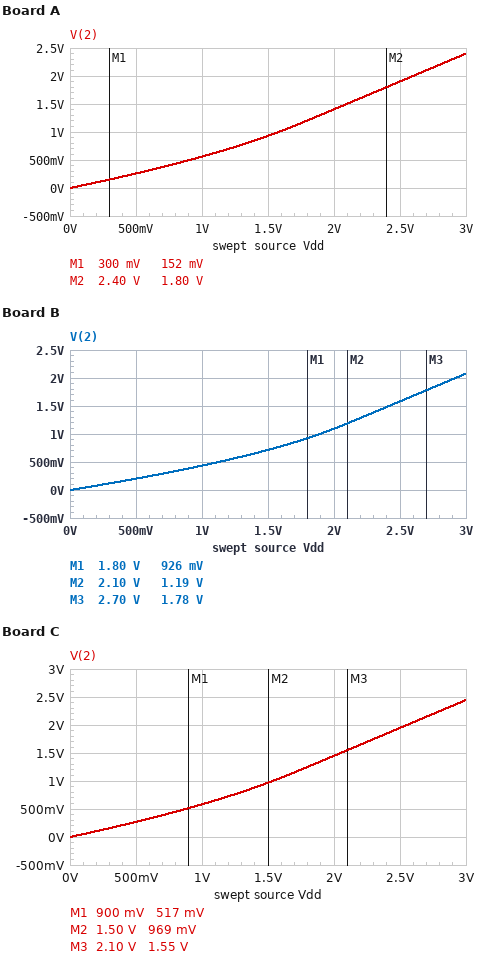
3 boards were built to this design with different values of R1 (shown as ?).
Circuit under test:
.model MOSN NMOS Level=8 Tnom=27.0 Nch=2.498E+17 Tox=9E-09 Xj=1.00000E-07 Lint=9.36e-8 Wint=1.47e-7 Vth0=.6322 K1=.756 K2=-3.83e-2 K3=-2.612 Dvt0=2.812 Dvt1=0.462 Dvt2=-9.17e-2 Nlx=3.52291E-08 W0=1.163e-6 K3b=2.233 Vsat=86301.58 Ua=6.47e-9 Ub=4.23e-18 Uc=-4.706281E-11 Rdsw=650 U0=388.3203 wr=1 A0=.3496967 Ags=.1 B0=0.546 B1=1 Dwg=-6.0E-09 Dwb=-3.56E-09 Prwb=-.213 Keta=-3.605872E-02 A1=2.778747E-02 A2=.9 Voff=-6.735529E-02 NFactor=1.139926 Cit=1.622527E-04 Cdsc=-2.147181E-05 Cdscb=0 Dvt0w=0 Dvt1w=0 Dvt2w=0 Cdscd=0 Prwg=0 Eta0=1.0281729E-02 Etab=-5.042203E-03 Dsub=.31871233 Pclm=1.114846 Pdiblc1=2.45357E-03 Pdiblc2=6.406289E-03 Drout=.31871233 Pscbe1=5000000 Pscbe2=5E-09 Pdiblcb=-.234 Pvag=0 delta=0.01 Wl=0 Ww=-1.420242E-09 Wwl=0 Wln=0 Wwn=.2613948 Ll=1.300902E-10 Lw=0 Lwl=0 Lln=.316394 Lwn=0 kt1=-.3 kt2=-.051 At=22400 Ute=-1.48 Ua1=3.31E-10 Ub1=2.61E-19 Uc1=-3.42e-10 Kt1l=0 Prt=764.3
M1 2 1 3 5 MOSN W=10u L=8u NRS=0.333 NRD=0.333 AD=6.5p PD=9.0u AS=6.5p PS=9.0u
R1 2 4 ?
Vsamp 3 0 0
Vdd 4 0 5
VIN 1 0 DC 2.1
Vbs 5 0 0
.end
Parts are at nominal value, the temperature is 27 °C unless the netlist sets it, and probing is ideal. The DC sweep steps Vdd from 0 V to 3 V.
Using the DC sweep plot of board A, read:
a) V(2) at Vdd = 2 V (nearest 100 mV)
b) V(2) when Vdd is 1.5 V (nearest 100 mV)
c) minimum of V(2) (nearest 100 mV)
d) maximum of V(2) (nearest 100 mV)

1.4 V
900 mV
0 V
2.4 V
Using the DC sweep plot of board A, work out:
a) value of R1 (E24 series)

13 kΩ
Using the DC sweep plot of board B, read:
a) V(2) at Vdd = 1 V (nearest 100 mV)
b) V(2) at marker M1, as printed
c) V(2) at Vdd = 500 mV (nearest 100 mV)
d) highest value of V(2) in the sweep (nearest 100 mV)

400 mV
926 mV
200 mV
2.1 V
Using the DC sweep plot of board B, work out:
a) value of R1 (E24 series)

20 kΩ
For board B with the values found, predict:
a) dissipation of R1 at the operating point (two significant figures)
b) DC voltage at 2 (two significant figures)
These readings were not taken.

43 µW
4.1 V
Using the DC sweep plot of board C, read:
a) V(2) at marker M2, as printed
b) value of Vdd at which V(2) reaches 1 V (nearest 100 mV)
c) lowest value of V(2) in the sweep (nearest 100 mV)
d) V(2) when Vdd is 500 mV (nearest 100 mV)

969 mV
1.5 V
0 V
300 mV
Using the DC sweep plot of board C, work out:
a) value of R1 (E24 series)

12 kΩ
